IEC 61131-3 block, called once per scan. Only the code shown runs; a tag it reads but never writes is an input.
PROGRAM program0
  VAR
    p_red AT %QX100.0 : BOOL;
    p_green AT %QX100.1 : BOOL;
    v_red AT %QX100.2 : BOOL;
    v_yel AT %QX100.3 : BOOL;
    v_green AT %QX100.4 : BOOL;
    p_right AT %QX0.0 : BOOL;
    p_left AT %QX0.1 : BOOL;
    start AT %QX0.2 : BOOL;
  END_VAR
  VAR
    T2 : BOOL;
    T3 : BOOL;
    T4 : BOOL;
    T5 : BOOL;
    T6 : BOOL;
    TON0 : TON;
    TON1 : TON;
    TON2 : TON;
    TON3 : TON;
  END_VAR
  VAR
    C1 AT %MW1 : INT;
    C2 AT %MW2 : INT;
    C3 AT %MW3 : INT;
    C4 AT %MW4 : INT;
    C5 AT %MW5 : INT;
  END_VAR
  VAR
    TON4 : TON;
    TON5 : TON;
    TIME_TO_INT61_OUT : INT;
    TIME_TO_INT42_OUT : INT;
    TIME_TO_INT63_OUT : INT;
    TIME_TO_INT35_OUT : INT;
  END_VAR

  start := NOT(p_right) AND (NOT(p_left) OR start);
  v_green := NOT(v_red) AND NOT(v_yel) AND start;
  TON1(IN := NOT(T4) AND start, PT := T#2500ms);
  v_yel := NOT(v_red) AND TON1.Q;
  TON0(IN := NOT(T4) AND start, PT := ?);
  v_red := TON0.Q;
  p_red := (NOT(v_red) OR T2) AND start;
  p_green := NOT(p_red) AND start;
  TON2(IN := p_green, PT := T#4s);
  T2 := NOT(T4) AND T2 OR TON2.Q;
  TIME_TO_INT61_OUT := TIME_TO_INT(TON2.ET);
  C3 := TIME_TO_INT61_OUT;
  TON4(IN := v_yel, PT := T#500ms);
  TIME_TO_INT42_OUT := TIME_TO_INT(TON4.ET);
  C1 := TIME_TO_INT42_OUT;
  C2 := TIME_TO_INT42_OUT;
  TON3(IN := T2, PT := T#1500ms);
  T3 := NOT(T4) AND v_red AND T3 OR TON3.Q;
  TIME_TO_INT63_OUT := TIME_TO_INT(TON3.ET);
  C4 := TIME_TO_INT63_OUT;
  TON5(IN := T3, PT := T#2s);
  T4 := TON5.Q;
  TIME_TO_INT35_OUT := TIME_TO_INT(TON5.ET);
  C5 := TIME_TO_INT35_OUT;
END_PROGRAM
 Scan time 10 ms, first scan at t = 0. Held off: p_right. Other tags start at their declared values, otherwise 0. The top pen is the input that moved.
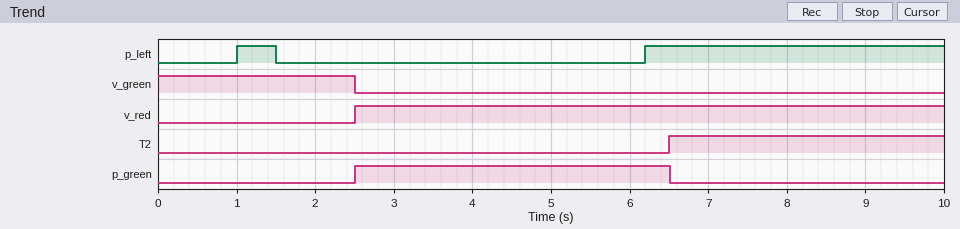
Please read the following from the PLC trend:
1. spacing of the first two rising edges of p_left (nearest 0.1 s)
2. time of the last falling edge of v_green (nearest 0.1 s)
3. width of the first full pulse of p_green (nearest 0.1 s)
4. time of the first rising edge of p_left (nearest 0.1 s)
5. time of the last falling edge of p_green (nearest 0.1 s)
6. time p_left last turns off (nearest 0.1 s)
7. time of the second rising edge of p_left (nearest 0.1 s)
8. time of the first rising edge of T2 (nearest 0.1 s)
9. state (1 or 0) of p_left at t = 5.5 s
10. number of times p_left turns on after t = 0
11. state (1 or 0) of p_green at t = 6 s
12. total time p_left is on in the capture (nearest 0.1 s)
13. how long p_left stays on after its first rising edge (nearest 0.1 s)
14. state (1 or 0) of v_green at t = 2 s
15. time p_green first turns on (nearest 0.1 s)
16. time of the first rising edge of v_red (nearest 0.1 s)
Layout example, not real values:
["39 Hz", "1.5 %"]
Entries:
["5.2 s", "2.5 s", "4.0 s", "1.0 s", "6.5 s", "1.5 s", "6.2 s", "6.5 s", "0", "2", "1", "4.3 s", "0.5 s", "1", "2.5 s", "2.5 s"]
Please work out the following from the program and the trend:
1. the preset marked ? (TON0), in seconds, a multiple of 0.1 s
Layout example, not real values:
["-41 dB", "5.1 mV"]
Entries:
["2.5 s"]
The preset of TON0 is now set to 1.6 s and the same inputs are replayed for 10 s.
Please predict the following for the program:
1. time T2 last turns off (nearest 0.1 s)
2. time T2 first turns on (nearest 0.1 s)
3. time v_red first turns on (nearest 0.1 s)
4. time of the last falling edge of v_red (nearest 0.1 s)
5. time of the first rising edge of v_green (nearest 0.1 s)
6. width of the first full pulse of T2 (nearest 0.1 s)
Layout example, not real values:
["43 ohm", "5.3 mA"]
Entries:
["9.1 s", "5.6 s", "1.6 s", "9.1 s", "9.1 s", "3.5 s"]
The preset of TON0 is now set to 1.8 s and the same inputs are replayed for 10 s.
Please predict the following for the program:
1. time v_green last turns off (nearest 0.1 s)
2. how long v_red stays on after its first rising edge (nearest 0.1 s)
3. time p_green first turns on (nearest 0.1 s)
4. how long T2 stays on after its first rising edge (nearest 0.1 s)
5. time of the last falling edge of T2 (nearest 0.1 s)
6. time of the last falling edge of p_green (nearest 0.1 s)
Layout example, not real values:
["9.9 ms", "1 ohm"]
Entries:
["1.8 s", "7.5 s", "1.8 s", "3.5 s", "9.3 s", "5.8 s"]
